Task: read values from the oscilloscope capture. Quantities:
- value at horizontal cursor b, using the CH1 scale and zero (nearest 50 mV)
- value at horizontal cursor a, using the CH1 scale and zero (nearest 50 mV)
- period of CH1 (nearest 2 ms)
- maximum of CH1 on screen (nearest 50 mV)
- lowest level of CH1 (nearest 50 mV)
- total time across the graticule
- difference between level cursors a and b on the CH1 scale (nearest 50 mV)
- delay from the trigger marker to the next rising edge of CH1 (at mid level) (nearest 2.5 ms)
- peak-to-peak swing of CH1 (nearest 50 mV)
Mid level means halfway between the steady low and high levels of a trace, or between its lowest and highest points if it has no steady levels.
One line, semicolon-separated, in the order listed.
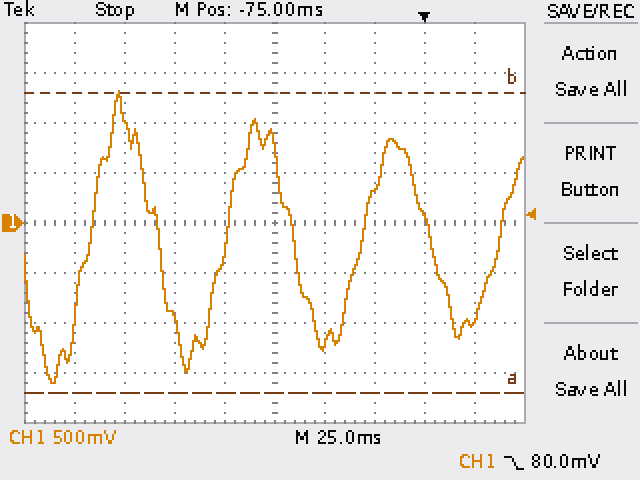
1.30 V; -1.70 V; 68 ms; 1.30 V; -1.60 V; 250 ms; 3.00 V; 37.5 ms; 2.90 V
